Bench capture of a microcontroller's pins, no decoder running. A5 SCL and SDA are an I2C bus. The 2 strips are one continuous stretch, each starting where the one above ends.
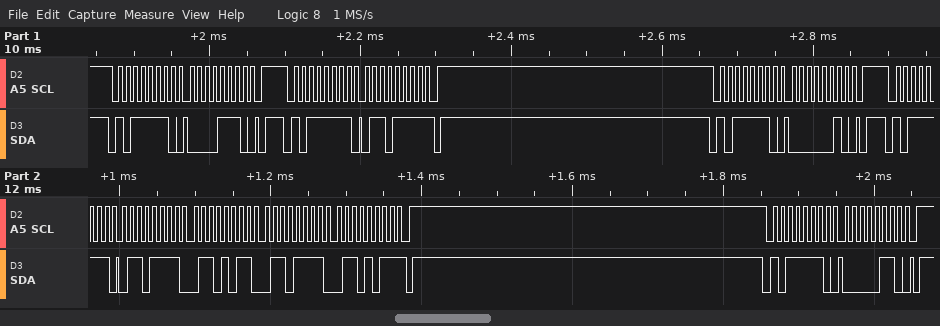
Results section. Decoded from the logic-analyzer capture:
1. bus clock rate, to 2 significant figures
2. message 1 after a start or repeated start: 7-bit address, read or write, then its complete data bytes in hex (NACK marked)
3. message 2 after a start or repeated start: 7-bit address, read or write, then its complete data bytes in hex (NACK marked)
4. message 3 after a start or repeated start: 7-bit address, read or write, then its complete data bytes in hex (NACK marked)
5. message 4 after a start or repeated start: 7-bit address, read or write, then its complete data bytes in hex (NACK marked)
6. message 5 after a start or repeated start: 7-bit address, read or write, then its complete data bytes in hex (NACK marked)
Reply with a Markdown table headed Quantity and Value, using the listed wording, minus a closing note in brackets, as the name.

| Quantity | Value |
|---|---|
| bus clock rate, to 2 significant figures | 100 kHz |
| message 1 after a start or repeated start: 7-bit address, read or write, then its complete data bytes in hex | 0x5F write: 0E |
| message 2 after a start or repeated start: 7-bit address, read or write, then its complete data bytes in hex | 0x5F read: 6F NACK |
| message 3 after a start or repeated start: 7-bit address, read or write, then its complete data bytes in hex | 0x5F write: 02 |
| message 4 after a start or repeated start: 7-bit address, read or write, then its complete data bytes in hex | 0x5F read: 6F 6B 6F 6B NACK |
| message 5 after a start or repeated start: 7-bit address, read or write, then its complete data bytes in hex | 0x5F write: 06 |
